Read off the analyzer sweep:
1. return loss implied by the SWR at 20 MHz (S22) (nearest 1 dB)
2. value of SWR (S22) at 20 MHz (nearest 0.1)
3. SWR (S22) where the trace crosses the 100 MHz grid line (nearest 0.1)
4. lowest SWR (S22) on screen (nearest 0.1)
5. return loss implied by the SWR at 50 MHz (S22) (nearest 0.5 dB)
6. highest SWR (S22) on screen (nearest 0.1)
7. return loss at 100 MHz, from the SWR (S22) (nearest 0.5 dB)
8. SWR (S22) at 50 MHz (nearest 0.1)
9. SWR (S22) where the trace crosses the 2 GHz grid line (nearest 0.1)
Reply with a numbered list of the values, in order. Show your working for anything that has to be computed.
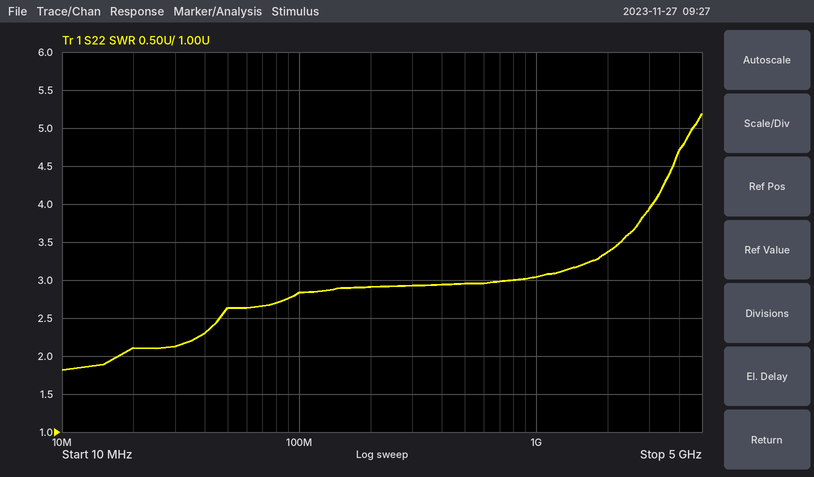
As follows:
1. −20 log10((2.1 − 1)/(2.1 + 1)) ≈ 9 dB
2. 2.1
3. 2.8
4. 1.8
5. −20 log10((2.6 − 1)/(2.6 + 1)) ≈ 7.0 dB
6. 5.2
7. −20 log10((2.8 − 1)/(2.8 + 1)) ≈ 6.5 dB
8. 2.6
9. 3.4
